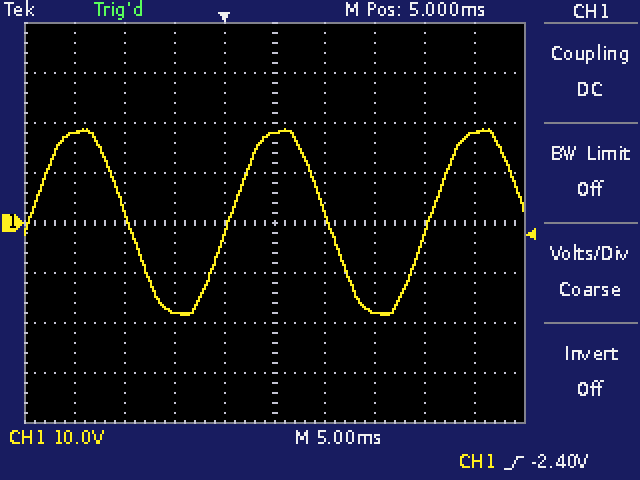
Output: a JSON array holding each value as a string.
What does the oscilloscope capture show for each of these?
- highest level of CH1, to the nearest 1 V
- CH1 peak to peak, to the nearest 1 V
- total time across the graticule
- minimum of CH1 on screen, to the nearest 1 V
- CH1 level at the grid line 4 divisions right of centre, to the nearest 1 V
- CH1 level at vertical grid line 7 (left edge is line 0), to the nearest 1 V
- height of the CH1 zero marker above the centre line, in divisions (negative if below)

["19 V", "37 V", "50 ms", "-18 V", "18 V", "-18 V", "0.0 div"]
